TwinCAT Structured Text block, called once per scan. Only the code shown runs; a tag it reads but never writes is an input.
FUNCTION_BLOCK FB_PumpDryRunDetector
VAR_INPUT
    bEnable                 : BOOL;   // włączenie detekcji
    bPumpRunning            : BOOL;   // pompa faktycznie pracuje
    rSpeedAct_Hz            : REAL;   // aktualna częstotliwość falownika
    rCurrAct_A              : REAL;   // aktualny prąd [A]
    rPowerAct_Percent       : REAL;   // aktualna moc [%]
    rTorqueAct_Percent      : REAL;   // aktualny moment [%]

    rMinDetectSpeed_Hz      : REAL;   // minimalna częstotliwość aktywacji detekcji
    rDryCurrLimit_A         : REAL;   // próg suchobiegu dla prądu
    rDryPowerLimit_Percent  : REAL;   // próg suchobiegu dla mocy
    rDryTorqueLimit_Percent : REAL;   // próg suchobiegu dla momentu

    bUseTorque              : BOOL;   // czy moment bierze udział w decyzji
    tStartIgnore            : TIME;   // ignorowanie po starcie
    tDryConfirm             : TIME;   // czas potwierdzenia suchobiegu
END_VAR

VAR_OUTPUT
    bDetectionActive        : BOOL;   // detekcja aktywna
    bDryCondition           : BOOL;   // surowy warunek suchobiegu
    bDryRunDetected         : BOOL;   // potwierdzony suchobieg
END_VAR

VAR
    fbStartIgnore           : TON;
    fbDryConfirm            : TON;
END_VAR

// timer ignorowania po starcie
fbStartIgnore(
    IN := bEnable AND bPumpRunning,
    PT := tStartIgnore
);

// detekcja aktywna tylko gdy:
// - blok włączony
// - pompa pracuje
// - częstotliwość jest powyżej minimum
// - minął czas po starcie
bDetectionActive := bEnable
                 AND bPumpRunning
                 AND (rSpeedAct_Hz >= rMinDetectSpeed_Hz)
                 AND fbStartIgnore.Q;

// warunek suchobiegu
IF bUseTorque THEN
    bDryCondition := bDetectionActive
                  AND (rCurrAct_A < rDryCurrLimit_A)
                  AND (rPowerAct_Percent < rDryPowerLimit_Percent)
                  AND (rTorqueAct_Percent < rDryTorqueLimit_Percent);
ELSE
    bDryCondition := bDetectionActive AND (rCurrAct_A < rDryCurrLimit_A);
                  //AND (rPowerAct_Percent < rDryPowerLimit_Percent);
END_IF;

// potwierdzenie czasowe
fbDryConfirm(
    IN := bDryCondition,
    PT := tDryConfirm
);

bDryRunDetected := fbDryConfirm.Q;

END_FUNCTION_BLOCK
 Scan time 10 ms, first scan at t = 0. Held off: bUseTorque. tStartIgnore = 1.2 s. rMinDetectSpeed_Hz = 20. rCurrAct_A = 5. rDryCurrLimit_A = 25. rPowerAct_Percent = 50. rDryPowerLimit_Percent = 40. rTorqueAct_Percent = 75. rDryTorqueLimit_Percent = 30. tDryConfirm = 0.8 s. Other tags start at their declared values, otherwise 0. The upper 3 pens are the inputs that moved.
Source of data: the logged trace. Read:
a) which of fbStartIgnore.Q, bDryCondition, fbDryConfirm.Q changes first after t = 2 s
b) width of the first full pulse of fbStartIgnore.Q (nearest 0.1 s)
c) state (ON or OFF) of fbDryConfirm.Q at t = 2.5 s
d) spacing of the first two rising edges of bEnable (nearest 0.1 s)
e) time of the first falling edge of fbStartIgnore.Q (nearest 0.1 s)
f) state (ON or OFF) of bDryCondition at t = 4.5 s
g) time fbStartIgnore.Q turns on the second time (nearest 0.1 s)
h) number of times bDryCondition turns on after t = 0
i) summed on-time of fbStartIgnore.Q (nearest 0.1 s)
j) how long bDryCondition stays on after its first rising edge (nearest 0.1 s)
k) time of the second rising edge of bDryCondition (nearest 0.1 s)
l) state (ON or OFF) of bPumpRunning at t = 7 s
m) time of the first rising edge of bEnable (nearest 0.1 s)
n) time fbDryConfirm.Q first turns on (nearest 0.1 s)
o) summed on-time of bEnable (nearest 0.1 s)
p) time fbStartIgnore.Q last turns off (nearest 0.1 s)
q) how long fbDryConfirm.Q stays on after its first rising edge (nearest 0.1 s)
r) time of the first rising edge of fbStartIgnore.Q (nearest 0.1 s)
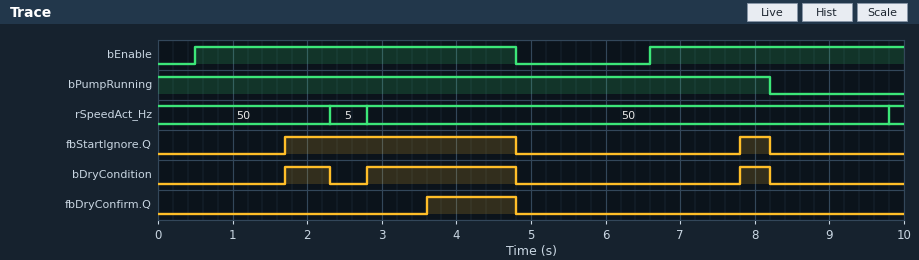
bDryCondition
3.1 s
OFF
6.1 s
4.8 s
ON
7.8 s
3
3.5 s
0.6 s
2.8 s
ON
0.5 s
3.6 s
7.7 s
8.2 s
1.2 s
1.7 s
